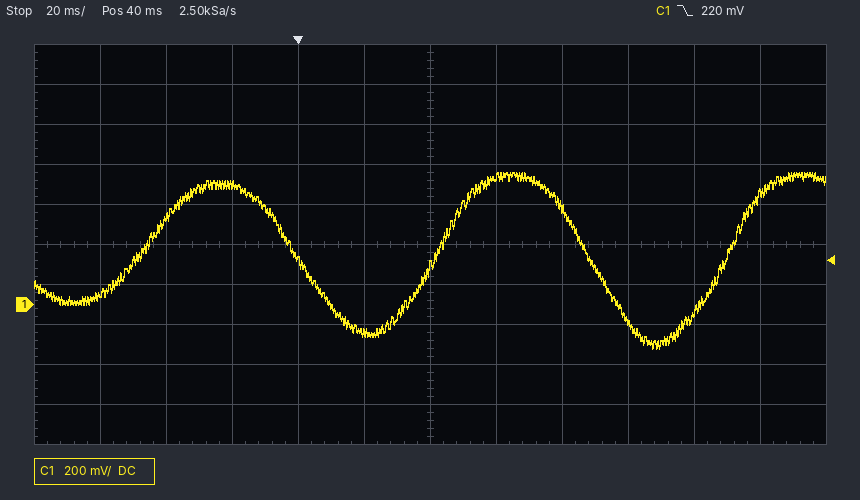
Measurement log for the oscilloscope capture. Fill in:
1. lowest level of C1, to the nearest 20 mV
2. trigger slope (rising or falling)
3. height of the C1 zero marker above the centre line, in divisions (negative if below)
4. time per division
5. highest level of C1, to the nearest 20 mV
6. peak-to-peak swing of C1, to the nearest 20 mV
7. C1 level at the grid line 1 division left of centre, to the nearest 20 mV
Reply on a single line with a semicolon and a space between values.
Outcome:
-220 mV; falling; -1.5 div; 20 ms; 660 mV; 880 mV; -140 mV
